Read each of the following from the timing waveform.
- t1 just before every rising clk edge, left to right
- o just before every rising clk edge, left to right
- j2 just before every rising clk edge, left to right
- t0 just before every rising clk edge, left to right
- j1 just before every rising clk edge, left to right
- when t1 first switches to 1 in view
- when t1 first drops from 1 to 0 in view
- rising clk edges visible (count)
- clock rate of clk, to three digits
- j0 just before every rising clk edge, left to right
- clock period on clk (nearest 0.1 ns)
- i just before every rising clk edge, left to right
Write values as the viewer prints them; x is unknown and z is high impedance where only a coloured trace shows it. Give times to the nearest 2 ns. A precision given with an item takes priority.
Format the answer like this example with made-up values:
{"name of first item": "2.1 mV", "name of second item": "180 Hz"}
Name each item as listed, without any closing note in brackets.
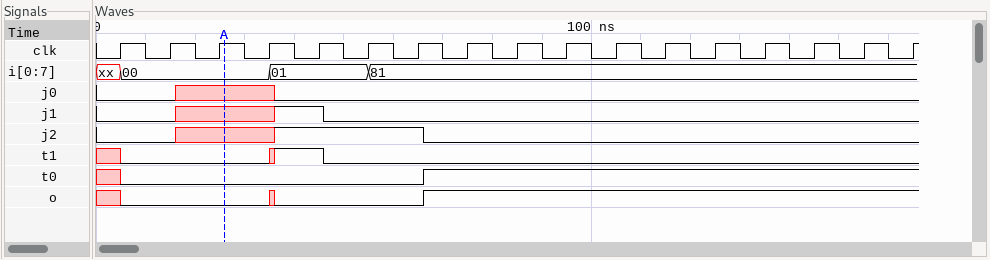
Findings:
{"t1 just before every rising clk edge, left to right": "x 0 0 0 1 0 0 0 0 0 0 0 0 0 0 0 0", "o just before every rising clk edge, left to right": "x 0 0 0 0 0 0 1 1 1 1 1 1 1 1 1 1", "j2 just before every rising clk edge, left to right": "0 0 x x 1 1 1 0 0 0 0 0 0 0 0 0 0", "t0 just before every rising clk edge, left to right": "x 0 0 0 0 0 0 1 1 1 1 1 1 1 1 1 1", "j1 just before every rising clk edge, left to right": "0 0 x x 1 0 0 0 0 0 0 0 0 0 0 0 0", "when t1 first switches to 1 in view": "36 ns", "when t1 first drops from 1 to 0 in view": "46 ns", "rising clk edges visible": "17", "clock rate of clk, to three digits": "100 MHz", "j0 just before every rising clk edge, left to right": "0 0 x x 0 0 0 0 0 0 0 0 0 0 0 0 0", "clock period on clk": "10 ns", "i just before every rising clk edge, left to right": "xx, 00, 00, 00, 01, 01, 81, 81, 81, 81, 81, 81, 81, 81, 81, 81, 81"}
